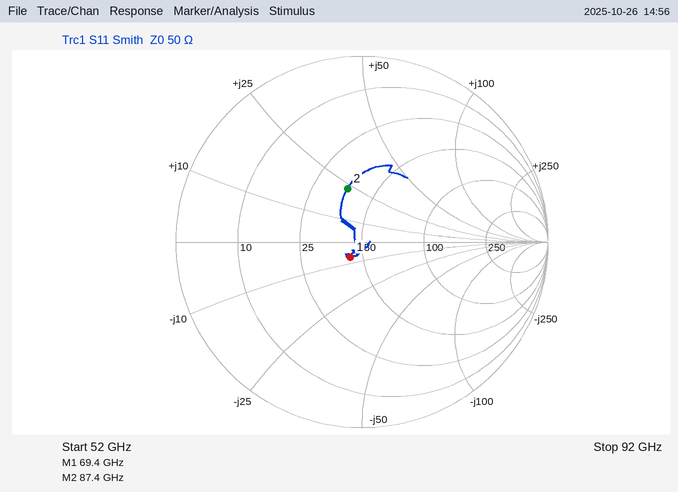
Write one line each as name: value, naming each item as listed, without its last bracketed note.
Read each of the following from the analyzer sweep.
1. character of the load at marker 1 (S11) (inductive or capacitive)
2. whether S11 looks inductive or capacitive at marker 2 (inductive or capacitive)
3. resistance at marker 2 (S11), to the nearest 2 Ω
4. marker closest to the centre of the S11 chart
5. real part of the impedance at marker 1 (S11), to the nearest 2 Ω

character of the load at marker 1 (S11): capacitive
whether S11 looks inductive or capacitive at marker 2: inductive
resistance at marker 2 (S11), to the nearest 2 Ω: 36 Ω
marker closest to the centre of the S11 chart: marker 1
real part of the impedance at marker 1 (S11), to the nearest 2 Ω: 44 Ω
